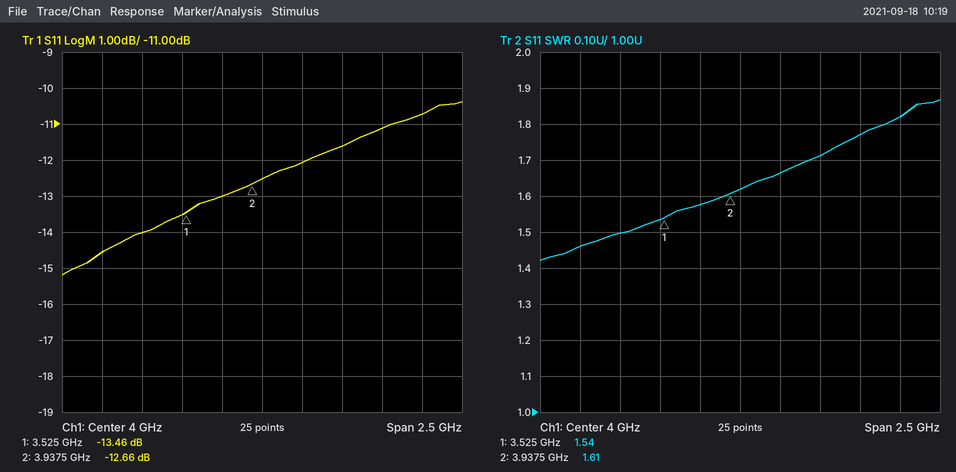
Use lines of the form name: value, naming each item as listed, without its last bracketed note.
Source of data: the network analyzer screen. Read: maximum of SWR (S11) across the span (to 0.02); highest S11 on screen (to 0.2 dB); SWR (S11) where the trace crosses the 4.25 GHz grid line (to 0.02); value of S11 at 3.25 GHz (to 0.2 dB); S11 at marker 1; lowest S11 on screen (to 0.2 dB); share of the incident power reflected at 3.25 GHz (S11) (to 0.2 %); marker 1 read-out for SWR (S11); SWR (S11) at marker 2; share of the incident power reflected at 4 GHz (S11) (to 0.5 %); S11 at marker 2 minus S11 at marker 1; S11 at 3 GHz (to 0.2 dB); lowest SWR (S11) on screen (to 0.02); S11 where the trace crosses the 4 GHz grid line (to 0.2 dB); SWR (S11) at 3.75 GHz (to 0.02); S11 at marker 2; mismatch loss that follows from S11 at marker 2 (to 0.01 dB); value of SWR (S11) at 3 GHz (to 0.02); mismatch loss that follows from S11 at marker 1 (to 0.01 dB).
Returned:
maximum of SWR (S11) across the span: 1.86
highest S11 on screen: -10.4 dB
SWR (S11) where the trace crosses the 4.25 GHz grid line: 1.66
value of S11 at 3.25 GHz: -14.0 dB
S11 at marker 1: -13.46 dB
lowest S11 on screen: -15.2 dB
share of the incident power reflected at 3.25 GHz (S11): 4.0 %
marker 1 read-out for SWR: 1.54
SWR (S11) at marker 2: 1.61
share of the incident power reflected at 4 GHz (S11): 5.5 %
S11 at marker 2 minus S11 at marker 1: 0.80 dB
S11 at 3 GHz: -14.6 dB
lowest SWR (S11) on screen: 1.42
S11 where the trace crosses the 4 GHz grid line: -12.6 dB
SWR (S11) at 3.75 GHz: 1.58
S11 at marker 2: -12.66 dB
mismatch loss that follows from S11 at marker 2: 0.24 dB
value of SWR (S11) at 3 GHz: 1.46
mismatch loss that follows from S11 at marker 1: 0.20 dB
